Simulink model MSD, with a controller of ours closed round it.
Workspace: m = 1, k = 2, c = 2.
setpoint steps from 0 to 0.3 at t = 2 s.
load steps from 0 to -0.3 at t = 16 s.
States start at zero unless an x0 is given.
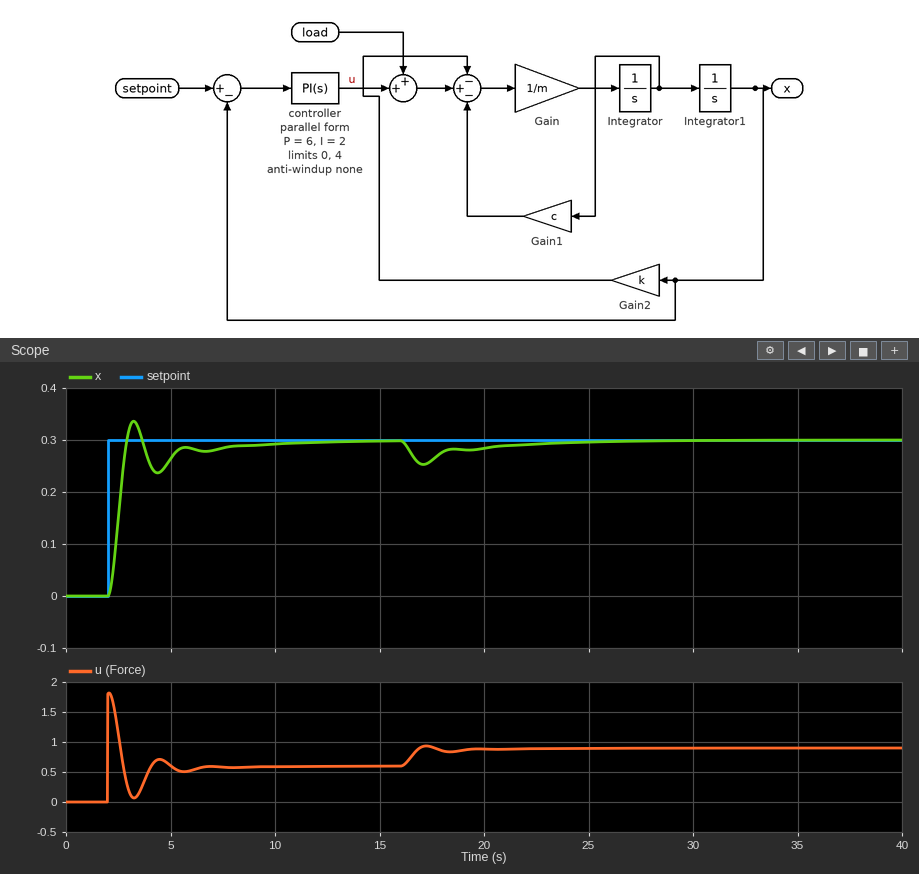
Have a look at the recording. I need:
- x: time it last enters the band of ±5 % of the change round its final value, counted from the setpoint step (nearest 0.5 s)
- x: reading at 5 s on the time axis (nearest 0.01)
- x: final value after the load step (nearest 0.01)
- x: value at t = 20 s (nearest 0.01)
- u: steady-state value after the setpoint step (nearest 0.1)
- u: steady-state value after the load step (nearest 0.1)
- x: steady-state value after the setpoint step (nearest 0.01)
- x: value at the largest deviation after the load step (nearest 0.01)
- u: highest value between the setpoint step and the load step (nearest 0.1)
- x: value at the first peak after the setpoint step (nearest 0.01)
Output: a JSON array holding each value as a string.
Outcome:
["5.5 s", "0.26", "0.30", "0.28", "0.6", "0.9", "0.30", "0.25", "1.8", "0.34"]
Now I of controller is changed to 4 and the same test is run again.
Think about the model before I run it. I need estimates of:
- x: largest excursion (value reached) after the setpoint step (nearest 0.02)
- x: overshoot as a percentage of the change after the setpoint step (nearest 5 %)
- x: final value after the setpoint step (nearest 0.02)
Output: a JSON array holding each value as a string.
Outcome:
["0.38", "25 %", "0.30"]
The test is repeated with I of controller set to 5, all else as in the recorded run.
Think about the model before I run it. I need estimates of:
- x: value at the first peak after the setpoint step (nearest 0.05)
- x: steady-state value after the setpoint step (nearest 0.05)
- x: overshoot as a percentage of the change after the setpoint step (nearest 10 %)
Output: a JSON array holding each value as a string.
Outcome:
["0.40", "0.30", "30 %"]
